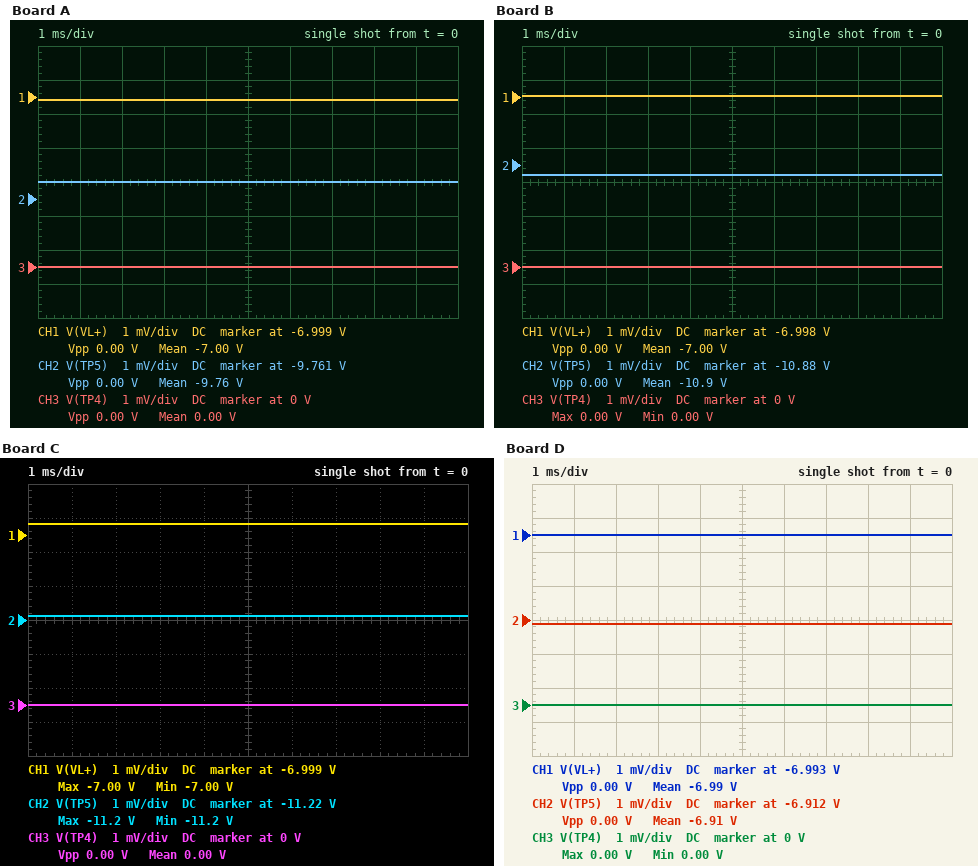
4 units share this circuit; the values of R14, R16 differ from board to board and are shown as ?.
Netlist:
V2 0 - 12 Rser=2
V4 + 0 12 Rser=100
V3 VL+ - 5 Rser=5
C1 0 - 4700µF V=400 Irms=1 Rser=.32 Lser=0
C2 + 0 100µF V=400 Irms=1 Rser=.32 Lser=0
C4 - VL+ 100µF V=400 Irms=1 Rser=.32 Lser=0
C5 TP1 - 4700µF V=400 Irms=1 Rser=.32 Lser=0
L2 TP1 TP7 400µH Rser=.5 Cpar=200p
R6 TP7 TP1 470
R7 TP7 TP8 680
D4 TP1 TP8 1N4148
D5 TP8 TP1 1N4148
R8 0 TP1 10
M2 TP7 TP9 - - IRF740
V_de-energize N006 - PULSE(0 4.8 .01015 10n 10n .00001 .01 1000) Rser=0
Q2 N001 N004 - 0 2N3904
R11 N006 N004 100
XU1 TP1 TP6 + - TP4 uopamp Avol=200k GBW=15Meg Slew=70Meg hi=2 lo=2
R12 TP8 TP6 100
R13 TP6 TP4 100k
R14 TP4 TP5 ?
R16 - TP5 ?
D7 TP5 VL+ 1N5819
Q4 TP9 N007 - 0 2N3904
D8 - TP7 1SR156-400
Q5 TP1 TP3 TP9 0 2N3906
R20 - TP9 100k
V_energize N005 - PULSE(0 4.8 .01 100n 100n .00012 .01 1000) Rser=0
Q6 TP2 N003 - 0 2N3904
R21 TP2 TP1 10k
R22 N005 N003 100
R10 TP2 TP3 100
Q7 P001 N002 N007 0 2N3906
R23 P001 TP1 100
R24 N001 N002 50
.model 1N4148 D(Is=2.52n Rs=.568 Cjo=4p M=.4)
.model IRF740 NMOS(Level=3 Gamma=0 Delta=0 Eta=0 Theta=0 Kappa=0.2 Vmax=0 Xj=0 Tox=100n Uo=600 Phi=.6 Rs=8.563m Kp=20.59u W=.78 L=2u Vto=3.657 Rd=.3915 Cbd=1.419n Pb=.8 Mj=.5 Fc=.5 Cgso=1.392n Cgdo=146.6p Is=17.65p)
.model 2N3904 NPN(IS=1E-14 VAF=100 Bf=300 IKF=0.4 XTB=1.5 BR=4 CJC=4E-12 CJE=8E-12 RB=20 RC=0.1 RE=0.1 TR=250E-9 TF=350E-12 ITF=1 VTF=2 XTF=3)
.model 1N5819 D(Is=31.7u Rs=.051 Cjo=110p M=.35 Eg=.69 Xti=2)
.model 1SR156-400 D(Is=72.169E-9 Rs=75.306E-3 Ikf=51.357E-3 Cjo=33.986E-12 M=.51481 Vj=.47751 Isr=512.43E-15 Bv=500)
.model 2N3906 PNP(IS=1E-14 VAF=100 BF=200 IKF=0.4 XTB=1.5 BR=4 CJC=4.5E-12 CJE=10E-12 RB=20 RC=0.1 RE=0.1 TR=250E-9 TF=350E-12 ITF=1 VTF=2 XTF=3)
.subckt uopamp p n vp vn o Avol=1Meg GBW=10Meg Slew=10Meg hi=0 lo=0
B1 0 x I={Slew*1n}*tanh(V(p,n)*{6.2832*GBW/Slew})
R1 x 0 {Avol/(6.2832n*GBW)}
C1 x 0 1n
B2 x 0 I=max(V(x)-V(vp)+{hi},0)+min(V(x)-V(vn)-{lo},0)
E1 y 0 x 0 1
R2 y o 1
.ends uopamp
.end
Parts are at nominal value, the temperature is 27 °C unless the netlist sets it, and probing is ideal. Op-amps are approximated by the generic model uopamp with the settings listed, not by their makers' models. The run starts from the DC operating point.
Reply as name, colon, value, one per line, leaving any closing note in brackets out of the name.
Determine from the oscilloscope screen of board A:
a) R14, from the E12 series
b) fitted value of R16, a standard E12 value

R14, from the E12 series: 18 kΩ
fitted value of R16, a standard E12 value: 3.9 kΩ
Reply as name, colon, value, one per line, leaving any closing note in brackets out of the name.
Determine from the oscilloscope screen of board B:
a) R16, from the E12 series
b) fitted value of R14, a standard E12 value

R16, from the E12 series: 1 kΩ
fitted value of R14, a standard E12 value: 10 kΩ
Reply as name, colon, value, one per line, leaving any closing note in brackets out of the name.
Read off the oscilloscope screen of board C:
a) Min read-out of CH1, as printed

Min read-out of CH1, as printed: -7.00 V
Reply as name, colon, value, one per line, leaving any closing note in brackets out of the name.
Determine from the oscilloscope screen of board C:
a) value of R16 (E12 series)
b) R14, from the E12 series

value of R16: 1 kΩ
R14, from the E12 series: 15 kΩ
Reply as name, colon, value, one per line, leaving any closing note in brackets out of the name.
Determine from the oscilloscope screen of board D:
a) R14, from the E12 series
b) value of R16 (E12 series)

R14, from the E12 series: 3.9 kΩ
value of R16: 4.7 kΩ
